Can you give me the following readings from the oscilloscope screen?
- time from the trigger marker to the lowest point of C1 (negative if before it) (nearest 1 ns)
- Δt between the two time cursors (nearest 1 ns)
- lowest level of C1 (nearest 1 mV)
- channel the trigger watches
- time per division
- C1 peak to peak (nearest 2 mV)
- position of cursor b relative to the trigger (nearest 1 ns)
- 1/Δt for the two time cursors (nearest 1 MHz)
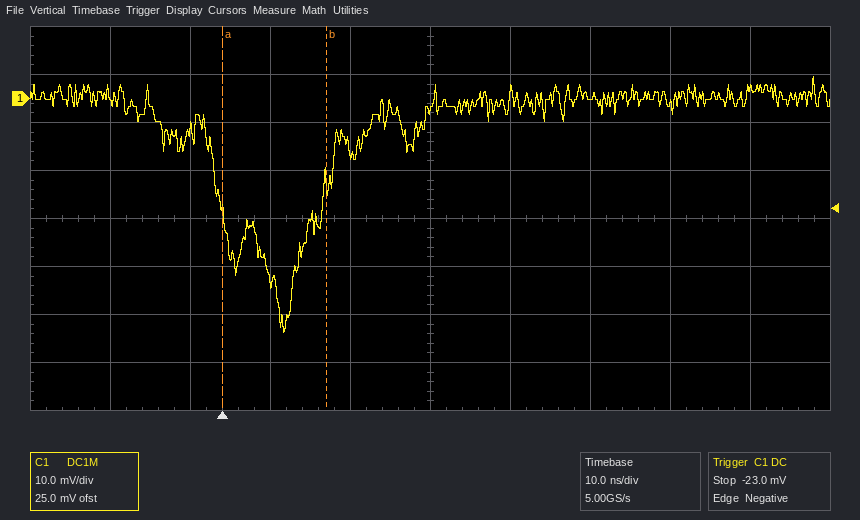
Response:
+8 ns
13 ns
-49 mV
C1
10 ns
54 mV
+13 ns
77 MHz
